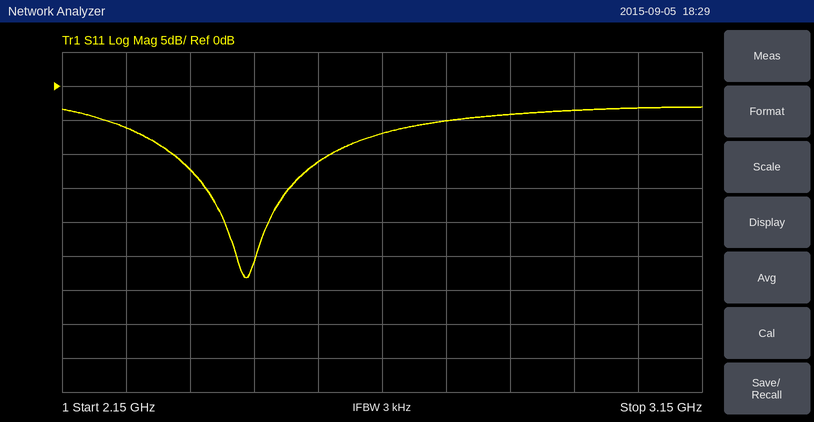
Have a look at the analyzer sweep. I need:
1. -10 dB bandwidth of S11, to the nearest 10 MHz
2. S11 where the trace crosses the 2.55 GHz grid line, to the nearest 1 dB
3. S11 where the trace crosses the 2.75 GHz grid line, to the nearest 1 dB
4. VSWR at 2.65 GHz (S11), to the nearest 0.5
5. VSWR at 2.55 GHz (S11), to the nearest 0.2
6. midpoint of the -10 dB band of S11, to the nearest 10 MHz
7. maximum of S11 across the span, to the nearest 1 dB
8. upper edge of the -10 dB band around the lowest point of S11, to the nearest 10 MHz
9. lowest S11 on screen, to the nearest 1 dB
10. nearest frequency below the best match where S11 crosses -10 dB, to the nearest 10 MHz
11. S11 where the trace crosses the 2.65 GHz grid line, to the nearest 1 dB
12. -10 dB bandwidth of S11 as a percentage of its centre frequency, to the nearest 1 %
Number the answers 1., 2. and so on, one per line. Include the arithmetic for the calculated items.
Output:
1. 2.57 GHz − 2.32 GHz = 250 MHz
2. -11 dB
3. -5 dB
4. |Γ| = 10^(-7/20) = 0.4467; VSWR = (1 + 0.4467)/(1 − 0.4467) ≈ 2.61, so 2.5 to the nearest 0.5
5. |Γ| = 10^(-11/20) = 0.2818; VSWR = (1 + 0.2818)/(1 − 0.2818) ≈ 1.8
6. 2.45 GHz
7. -3 dB
8. 2.57 GHz
9. -28 dB
10. 2.32 GHz
11. -7 dB
12. 250 MHz / 2.445 GHz ≈ 10 %
